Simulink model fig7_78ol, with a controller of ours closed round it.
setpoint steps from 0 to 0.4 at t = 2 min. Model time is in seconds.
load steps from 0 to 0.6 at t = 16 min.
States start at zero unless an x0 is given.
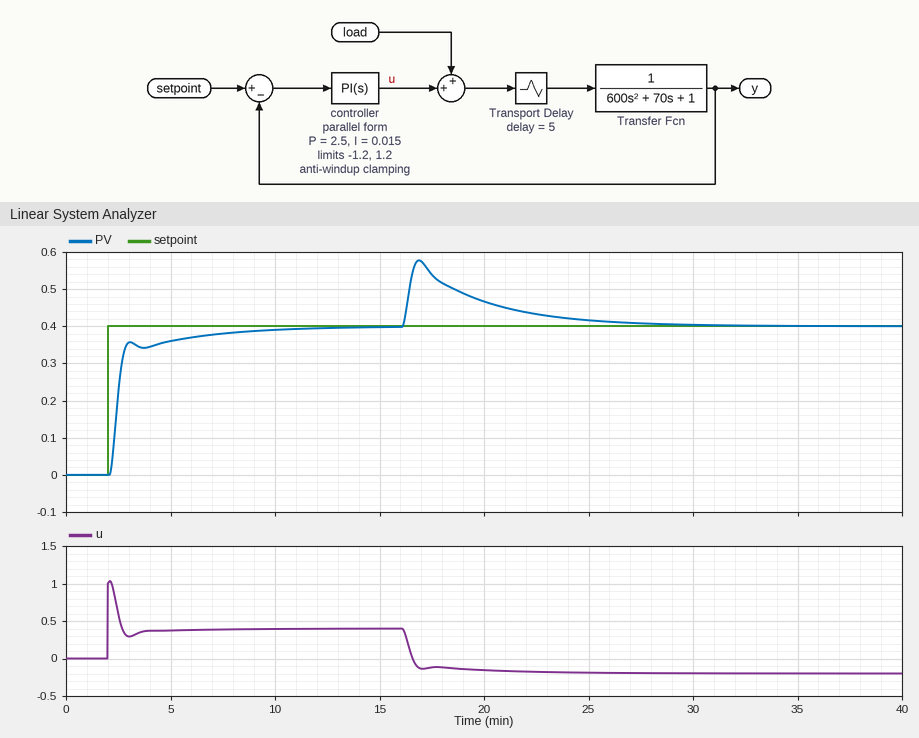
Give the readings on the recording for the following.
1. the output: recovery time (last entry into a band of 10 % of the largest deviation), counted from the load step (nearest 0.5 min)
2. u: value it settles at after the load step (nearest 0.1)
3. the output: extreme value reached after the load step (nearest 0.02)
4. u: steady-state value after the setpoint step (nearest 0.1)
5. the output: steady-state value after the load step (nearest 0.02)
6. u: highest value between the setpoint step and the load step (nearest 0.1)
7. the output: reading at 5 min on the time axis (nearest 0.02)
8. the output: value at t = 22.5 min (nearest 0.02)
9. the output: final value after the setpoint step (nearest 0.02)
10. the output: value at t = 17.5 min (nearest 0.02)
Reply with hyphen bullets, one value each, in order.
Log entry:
- 8.5 min
- -0.2
- 0.58
- 0.4
- 0.40
- 1.0
- 0.36
- 0.44
- 0.40
- 0.54
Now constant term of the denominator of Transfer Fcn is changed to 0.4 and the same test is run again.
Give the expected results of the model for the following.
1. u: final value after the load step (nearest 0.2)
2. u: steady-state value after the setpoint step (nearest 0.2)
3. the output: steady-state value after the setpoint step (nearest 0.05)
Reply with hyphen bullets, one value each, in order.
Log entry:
- -0.4
- 0.2
- 0.40
